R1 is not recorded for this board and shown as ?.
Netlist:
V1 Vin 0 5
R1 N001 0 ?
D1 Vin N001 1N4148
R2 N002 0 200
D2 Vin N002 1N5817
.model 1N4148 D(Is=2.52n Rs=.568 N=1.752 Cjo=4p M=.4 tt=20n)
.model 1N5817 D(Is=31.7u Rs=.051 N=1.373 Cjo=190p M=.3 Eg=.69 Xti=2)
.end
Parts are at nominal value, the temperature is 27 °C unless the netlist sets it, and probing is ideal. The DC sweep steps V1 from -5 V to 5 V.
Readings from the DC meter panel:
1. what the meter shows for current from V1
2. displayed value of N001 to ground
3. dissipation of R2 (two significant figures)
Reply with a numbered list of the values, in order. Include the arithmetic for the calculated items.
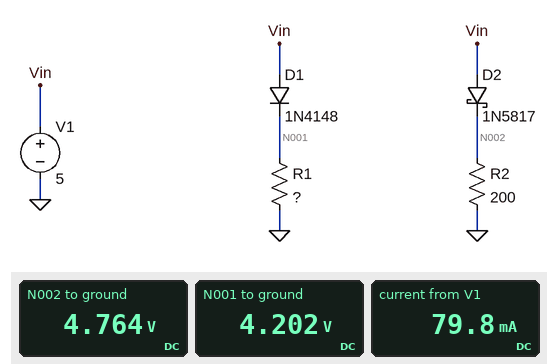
1. 79.8 mA
2. 4.202 V
3. (4.764 V)^2 / 200 Ω = 110 mW
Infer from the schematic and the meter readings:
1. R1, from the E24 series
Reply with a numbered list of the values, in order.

1. 75 Ω
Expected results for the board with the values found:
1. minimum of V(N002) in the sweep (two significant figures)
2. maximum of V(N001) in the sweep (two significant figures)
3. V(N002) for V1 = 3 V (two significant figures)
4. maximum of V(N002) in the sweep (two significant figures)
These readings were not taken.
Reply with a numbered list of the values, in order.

1. -6.3 mV
2. 4.2 V
3. 2.8 V
4. 4.8 V
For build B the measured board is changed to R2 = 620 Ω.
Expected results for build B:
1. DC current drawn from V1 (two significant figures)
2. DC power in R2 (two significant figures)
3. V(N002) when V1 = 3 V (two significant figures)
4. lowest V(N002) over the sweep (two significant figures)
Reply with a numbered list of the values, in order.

1. 64 mA
2. 37 mW
3. 2.8 V
4. -20 mV
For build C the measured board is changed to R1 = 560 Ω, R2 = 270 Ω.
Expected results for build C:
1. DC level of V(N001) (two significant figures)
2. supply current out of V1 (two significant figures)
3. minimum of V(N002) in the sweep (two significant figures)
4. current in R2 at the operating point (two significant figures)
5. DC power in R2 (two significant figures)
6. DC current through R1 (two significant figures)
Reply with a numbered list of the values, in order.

1. 4.3 V
2. 25 mA
3. -8.6 mV
4. 18 mA
5. 84 mW
6. 7.7 mA
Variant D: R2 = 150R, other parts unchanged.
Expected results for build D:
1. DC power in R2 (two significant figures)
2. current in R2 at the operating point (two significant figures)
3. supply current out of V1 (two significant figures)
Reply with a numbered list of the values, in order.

1. 150 mW
2. 32 mA
3. 88 mA
